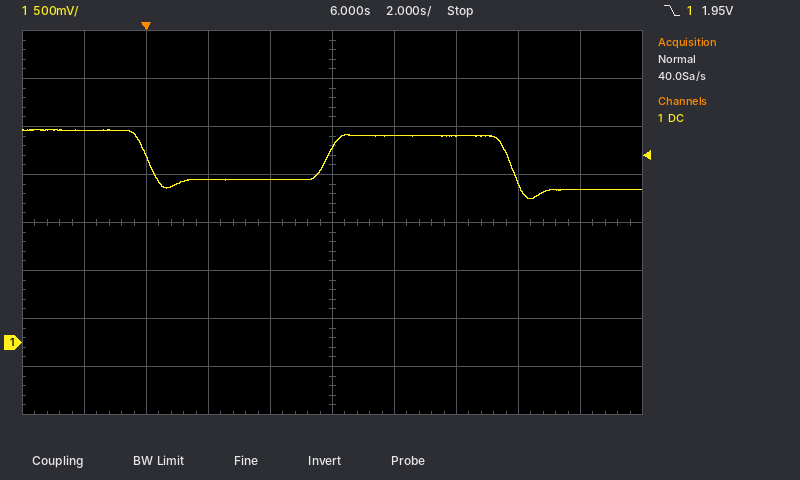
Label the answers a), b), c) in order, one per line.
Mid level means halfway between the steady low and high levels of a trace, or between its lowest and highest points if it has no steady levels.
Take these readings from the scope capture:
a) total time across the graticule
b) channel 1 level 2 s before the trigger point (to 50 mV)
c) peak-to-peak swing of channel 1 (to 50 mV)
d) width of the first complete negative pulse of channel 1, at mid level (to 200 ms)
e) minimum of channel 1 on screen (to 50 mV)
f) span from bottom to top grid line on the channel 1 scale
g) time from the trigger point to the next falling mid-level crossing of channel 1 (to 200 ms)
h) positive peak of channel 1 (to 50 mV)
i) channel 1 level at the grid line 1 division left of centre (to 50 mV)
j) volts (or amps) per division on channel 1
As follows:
a) 20 s
b) 2.20 V
c) 700 mV
d) 5.6 s
e) 1.50 V
f) 4 V
g) 200 ms
h) 2.20 V
i) 1.70 V
j) 500 mV
